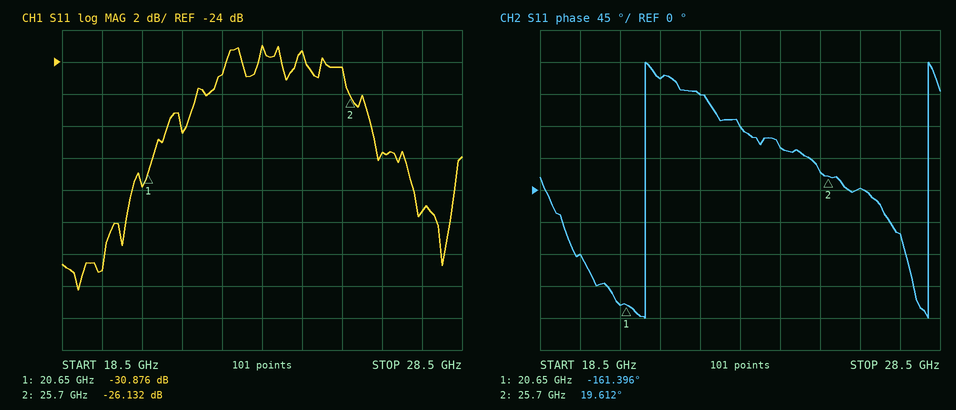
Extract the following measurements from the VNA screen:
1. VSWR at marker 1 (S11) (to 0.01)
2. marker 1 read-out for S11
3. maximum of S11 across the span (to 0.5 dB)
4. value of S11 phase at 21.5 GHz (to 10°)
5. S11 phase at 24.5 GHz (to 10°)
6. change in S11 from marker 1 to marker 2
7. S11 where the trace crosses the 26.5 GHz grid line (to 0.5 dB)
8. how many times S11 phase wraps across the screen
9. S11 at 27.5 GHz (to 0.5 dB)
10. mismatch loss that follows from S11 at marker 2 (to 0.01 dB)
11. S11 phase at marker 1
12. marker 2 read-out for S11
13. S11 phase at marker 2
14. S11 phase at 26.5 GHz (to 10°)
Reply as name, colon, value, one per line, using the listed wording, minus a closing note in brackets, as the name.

VSWR at marker 1 (S11): 1.06
marker 1 read-out for S11: -30.876 dB
maximum of S11 across the span: -23.0 dB
value of S11 phase at 21.5 GHz: 160°
S11 phase at 24.5 GHz: 60°
change in S11 from marker 1 to marker 2: 4.744 dB
S11 where the trace crosses the 26.5 GHz grid line: -29.5 dB
how many times S11 phase wraps across the screen: 2
S11 at 27.5 GHz: -33.5 dB
mismatch loss that follows from S11 at marker 2: 0.01 dB
S11 phase at marker 1: -161.396°
marker 2 read-out for S11: -26.132 dB
S11 phase at marker 2: 19.612°
S11 phase at 26.5 GHz: 0°
